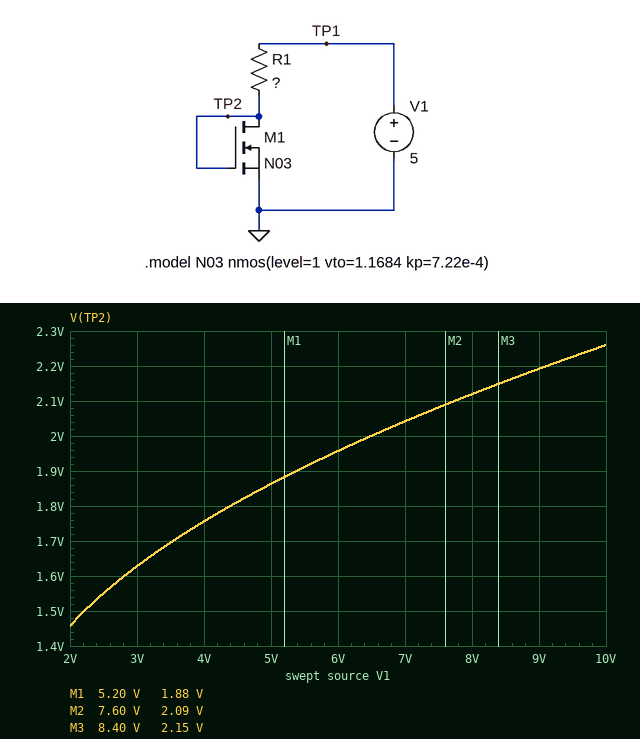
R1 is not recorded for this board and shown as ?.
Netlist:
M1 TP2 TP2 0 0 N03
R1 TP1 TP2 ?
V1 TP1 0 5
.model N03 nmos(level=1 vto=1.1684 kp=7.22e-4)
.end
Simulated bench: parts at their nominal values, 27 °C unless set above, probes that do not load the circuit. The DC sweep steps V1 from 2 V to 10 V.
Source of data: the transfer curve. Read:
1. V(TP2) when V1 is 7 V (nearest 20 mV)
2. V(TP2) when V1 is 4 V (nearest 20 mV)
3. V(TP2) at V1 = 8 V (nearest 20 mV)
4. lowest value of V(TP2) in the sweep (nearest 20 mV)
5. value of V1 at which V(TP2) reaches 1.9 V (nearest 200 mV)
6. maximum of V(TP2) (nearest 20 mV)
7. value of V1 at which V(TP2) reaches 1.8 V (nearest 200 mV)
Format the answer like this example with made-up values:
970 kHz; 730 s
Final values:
2.04 V; 1.76 V; 2.12 V; 1.46 V; 5.4 V; 2.26 V; 4.4 V
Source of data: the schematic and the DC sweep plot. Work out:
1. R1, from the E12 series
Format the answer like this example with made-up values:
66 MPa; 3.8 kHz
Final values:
18 kΩ
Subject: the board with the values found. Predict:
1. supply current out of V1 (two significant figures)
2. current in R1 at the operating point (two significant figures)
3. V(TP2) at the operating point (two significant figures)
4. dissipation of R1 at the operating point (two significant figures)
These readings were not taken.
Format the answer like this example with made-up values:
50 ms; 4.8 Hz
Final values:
170 µA; 170 µA; 1.9 V; 550 µW
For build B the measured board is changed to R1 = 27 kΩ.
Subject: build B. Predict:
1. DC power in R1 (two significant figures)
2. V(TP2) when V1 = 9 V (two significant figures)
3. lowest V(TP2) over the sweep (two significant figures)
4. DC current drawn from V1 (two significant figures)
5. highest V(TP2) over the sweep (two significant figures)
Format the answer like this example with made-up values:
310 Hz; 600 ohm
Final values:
390 µW; 2.0 V; 1.4 V; 120 µA; 2.1 V
